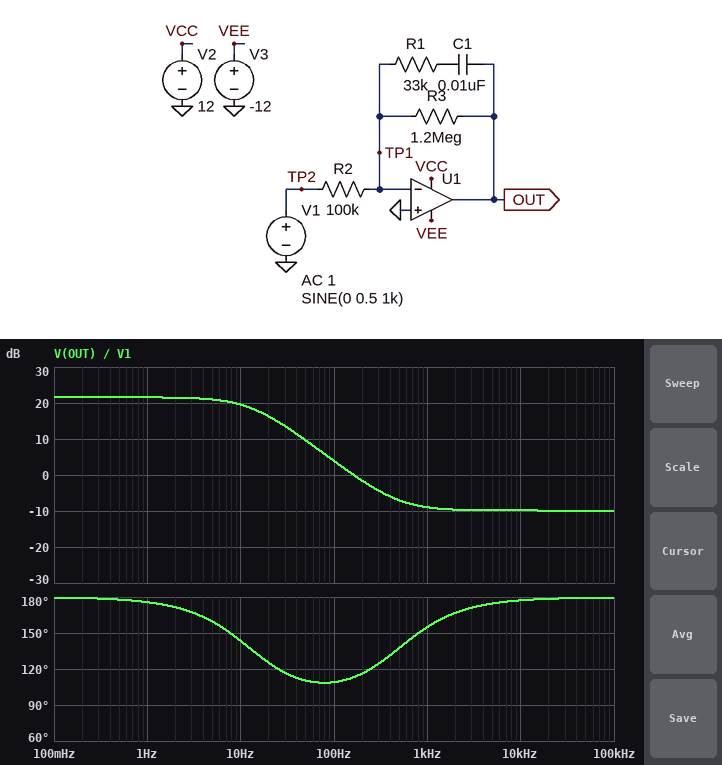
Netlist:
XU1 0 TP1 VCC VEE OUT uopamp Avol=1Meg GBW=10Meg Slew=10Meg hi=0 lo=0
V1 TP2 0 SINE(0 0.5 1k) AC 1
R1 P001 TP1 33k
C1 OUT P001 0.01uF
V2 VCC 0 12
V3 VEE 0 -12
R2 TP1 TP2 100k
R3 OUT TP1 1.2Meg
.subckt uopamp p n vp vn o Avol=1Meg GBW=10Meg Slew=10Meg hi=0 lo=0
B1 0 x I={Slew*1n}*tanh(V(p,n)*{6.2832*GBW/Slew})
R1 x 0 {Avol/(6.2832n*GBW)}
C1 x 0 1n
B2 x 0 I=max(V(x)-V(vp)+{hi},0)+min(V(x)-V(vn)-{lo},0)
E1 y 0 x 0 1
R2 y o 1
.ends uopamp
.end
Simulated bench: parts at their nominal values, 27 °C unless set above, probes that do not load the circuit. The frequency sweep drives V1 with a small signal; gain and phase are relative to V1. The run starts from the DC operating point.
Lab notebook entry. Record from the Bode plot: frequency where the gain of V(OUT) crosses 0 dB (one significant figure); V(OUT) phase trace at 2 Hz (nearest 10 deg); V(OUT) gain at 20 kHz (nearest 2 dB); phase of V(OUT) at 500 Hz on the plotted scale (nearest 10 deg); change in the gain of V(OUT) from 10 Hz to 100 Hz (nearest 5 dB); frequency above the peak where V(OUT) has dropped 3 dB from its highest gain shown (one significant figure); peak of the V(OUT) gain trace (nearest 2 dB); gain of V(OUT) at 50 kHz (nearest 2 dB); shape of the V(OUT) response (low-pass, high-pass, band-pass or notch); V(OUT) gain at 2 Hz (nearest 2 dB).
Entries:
200 Hz
170 deg
-10 dB
140 deg
-15 dB
10 Hz
22 dB
-10 dB
low-pass
22 dB
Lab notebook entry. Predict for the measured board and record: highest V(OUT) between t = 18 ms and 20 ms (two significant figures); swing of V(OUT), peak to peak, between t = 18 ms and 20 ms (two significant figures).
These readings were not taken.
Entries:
160 mV
360 mV
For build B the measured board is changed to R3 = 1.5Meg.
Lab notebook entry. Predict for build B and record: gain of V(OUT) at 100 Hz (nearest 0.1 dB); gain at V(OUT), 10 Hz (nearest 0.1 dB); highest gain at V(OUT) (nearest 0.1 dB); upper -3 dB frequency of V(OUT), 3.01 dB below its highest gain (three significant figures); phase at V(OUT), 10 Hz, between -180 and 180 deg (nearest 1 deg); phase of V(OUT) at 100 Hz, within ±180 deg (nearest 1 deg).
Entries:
4.0 dB
20.7 dB
23.5 dB
10.4 Hz
137 deg
108 deg
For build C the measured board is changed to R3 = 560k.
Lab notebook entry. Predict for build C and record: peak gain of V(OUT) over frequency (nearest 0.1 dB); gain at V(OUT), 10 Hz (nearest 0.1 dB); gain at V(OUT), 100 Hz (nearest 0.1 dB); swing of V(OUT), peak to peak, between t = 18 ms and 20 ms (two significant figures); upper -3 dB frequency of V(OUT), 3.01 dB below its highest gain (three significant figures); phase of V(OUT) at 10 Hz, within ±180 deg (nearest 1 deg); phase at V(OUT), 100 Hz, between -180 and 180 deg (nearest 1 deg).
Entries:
15.0 dB
14.4 dB
3.4 dB
350 mV
26.9 Hz
161 deg
117 deg
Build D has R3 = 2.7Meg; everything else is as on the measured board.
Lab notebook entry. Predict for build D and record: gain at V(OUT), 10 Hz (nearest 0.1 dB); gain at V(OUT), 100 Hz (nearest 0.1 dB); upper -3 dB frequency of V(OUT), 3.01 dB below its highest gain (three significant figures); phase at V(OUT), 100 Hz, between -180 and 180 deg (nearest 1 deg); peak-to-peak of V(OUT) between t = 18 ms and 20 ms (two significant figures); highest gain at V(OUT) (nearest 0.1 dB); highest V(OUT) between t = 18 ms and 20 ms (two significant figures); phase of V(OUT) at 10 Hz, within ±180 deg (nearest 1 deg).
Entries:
22.7 dB
4.1 dB
5.82 Hz
105 deg
360 mV
28.6 dB
140 mV
121 deg
